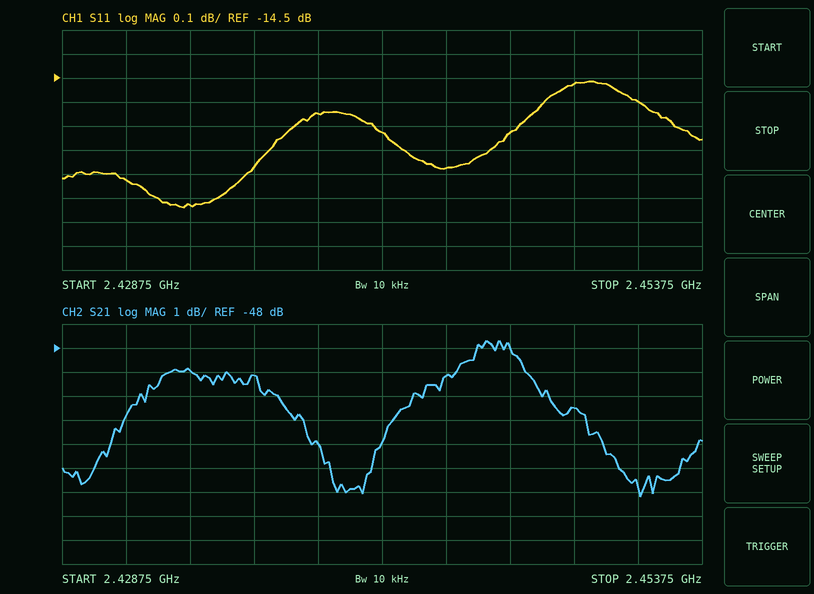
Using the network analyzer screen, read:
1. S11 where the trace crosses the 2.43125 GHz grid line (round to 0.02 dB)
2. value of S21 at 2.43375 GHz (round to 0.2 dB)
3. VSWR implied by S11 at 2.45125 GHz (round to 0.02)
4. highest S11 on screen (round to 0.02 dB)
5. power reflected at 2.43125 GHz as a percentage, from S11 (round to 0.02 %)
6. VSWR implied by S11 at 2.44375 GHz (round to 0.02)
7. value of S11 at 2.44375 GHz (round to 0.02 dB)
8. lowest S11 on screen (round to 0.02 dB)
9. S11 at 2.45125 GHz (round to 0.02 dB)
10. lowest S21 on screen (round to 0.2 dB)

-14.92 dB
-49.0 dB
1.46
-14.52 dB
3.22 %
1.44
-14.88 dB
-15.04 dB
-14.60 dB
-54.2 dB
